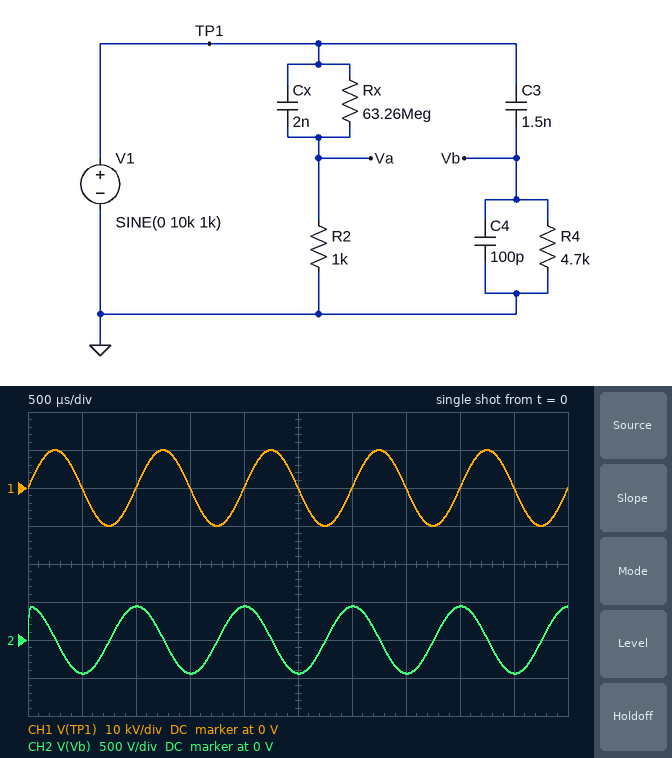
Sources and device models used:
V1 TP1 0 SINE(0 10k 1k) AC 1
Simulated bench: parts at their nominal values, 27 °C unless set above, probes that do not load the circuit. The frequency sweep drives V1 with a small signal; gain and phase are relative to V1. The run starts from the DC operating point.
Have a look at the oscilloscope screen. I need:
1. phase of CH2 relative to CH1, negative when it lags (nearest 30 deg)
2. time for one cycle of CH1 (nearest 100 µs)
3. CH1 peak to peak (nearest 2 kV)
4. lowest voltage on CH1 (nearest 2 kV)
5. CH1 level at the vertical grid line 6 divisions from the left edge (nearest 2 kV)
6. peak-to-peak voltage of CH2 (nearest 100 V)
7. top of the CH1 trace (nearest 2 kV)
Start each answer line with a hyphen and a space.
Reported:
- 90 deg
- 1.0 ms
- 20 kV
- -10 kV
- 0 V
- 900 V
- 10 kV
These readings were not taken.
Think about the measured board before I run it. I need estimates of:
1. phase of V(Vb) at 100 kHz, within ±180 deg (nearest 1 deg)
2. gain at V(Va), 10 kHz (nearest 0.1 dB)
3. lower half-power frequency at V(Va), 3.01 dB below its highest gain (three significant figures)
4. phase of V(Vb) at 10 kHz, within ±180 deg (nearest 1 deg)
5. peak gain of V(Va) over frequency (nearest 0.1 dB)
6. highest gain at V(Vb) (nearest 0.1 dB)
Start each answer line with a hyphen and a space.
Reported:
- 12 deg
- -18.1 dB
- 79.6 kHz
- 65 deg
- 0 dB
- -0.6 dB
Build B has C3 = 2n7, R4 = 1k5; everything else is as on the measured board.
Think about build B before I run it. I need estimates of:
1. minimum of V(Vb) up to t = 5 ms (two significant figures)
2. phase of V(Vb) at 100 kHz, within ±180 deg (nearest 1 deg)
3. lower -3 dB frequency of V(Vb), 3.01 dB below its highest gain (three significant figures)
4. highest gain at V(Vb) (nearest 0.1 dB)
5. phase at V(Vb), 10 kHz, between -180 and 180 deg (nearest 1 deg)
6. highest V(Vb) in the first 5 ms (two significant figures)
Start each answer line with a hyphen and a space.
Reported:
- -250 V
- 21 deg
- 37.9 kHz
- -0.3 dB
- 75 deg
- 250 V
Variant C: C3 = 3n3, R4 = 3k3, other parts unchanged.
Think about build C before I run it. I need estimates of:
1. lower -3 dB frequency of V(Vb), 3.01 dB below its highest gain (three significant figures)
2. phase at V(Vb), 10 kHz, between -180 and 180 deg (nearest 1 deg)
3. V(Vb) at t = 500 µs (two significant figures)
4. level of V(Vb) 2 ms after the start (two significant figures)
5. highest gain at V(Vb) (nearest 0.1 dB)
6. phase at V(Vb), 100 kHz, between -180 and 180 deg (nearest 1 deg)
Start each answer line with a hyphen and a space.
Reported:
- 14.2 kHz
- 55 deg
- -680 V
- 680 V
- -0.3 dB
- 8 deg
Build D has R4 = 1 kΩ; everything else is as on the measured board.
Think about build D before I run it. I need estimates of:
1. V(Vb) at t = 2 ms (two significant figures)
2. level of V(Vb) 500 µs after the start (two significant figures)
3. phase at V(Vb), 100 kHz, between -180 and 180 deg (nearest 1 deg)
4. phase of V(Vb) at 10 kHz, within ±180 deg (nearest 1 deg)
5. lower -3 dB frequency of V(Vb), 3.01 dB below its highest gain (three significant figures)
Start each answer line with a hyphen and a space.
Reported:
- 94 V
- -94 V
- 45 deg
- 84 deg
- 99.5 kHz
